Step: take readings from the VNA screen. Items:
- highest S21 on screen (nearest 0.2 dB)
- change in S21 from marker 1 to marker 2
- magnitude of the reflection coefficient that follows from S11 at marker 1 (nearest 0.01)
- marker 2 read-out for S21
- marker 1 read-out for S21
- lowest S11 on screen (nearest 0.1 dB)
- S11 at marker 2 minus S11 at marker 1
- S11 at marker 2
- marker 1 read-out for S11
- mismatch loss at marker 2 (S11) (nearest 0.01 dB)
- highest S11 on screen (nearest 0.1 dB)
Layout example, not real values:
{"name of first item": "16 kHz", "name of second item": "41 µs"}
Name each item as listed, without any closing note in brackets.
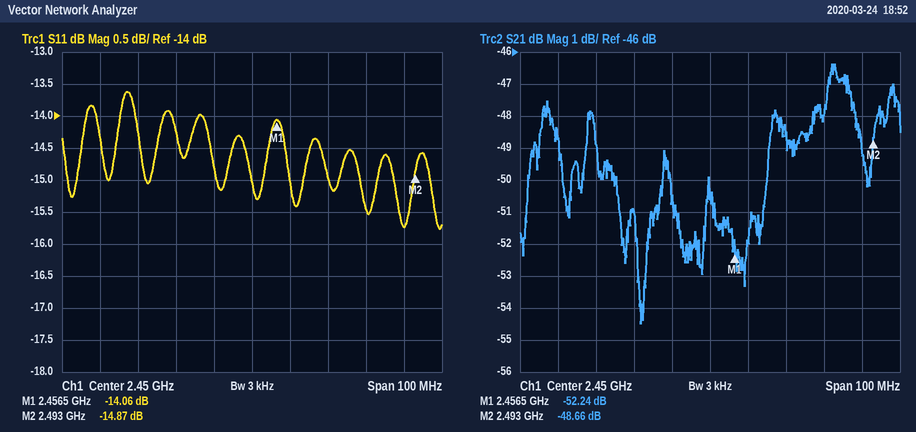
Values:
{"highest S21 on screen": "-46.4 dB", "change in S21 from marker 1 to marker 2": "3.58 dB", "magnitude of the reflection coefficient that follows from S11 at marker 1": "0.20", "marker 2 read-out for S21": "-48.66 dB", "marker 1 read-out for S21": "-52.24 dB", "lowest S11 on screen": "-15.8 dB", "S11 at marker 2 minus S11 at marker 1": "-0.81 dB", "S11 at marker 2": "-14.87 dB", "marker 1 read-out for S11": "-14.06 dB", "mismatch loss at marker 2 (S11)": "0.14 dB", "highest S11 on screen": "-13.6 dB"}
